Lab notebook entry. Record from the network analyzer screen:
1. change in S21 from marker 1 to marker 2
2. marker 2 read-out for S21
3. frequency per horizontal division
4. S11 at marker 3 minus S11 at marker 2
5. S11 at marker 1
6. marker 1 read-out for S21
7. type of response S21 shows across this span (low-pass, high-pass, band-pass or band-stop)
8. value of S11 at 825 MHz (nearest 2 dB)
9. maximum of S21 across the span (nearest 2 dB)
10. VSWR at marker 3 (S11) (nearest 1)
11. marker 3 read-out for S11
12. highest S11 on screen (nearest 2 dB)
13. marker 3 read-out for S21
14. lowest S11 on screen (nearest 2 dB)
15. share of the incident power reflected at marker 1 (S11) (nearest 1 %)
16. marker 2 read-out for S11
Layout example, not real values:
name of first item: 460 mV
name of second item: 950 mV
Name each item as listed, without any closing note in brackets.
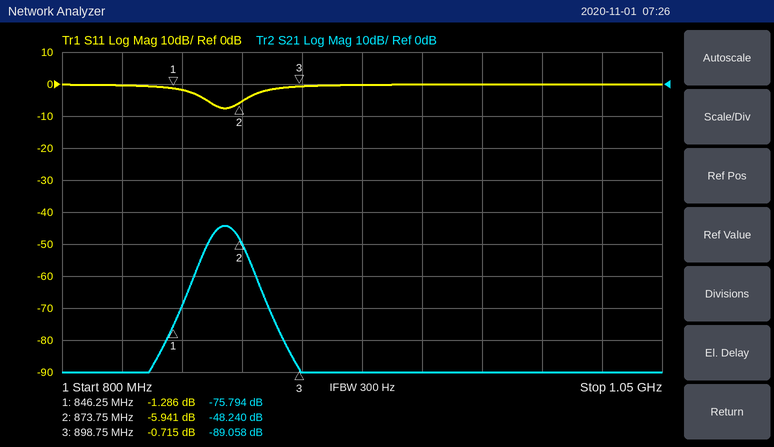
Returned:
change in S21 from marker 1 to marker 2: 27.554 dB
marker 2 read-out for S21: -48.240 dB
frequency per horizontal division: 25 MHz
S11 at marker 3 minus S11 at marker 2: 5.226 dB
S11 at marker 1: -1.286 dB
marker 1 read-out for S21: -75.794 dB
type of response S21 shows across this span: band-pass
value of S11 at 825 MHz: 0 dB
maximum of S21 across the span: -44 dB
VSWR at marker 3 (S11): 24
marker 3 read-out for S11: -0.715 dB
highest S11 on screen: 0 dB
marker 3 read-out for S21: -89.058 dB
lowest S11 on screen: -8 dB
share of the incident power reflected at marker 1 (S11): 74 %
marker 2 read-out for S11: -5.941 dB
